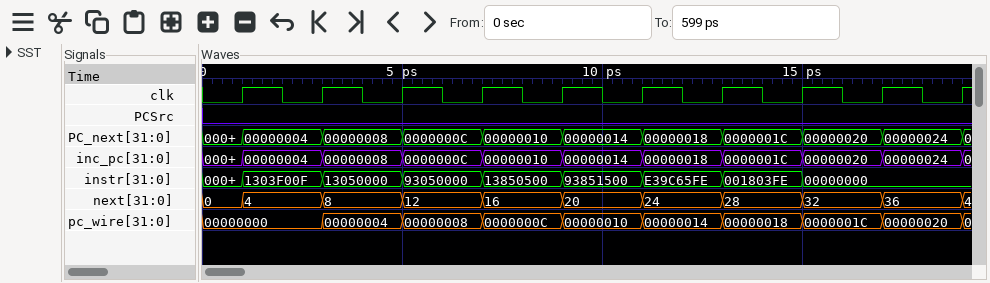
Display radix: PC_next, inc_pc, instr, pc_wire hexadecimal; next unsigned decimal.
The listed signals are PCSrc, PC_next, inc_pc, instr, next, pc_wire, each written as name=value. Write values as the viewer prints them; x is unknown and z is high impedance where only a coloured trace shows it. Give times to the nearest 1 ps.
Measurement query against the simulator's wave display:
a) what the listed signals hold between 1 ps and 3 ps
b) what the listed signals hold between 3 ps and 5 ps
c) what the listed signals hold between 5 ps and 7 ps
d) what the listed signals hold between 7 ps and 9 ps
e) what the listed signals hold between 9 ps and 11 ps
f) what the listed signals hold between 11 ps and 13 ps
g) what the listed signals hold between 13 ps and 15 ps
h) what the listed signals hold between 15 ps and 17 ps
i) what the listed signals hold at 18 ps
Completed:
PCSrc=0, PC_next=00000004, inc_pc=00000004, instr=1303F00F, next=4, pc_wire=00000000
PCSrc=0, PC_next=00000008, inc_pc=00000008, instr=13050000, next=8, pc_wire=00000004
PCSrc=0, PC_next=0000000C, inc_pc=0000000C, instr=93050000, next=12, pc_wire=00000008
PCSrc=0, PC_next=00000010, inc_pc=00000010, instr=13850500, next=16, pc_wire=0000000C
PCSrc=0, PC_next=00000014, inc_pc=00000014, instr=93851500, next=20, pc_wire=00000010
PCSrc=0, PC_next=00000018, inc_pc=00000018, instr=E39C65FE, next=24, pc_wire=00000014
PCSrc=0, PC_next=0000001C, inc_pc=0000001C, instr=001803FE, next=28, pc_wire=00000018
PCSrc=0, PC_next=00000020, inc_pc=00000020, instr=00000000, next=32, pc_wire=0000001C
PCSrc=0, PC_next=00000024, inc_pc=00000024, instr=00000000, next=36, pc_wire=00000020
